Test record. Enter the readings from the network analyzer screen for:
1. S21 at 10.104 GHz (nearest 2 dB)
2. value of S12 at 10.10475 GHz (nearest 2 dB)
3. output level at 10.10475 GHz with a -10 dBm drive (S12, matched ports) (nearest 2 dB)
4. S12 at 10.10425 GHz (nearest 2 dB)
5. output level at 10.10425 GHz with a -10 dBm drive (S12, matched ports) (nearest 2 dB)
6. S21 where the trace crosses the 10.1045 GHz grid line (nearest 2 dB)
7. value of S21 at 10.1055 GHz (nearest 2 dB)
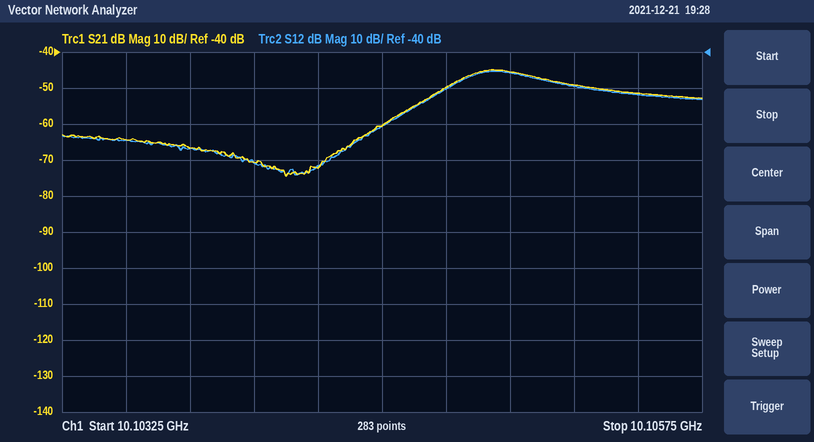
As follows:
-70 dB
-50 dB
-60 dBm
-72 dB
-82 dBm
-60 dB
-52 dB
